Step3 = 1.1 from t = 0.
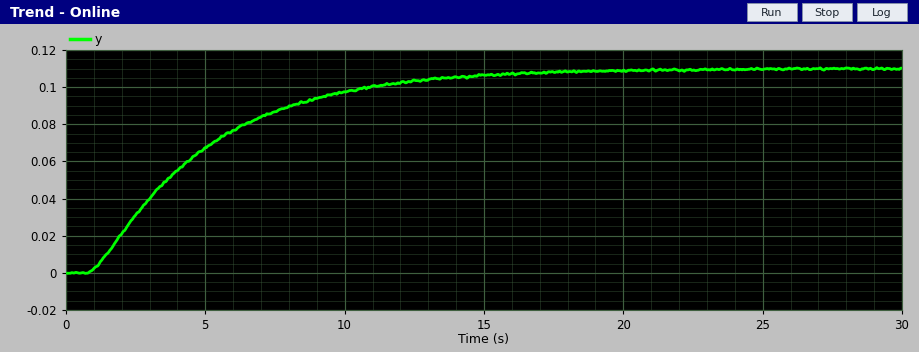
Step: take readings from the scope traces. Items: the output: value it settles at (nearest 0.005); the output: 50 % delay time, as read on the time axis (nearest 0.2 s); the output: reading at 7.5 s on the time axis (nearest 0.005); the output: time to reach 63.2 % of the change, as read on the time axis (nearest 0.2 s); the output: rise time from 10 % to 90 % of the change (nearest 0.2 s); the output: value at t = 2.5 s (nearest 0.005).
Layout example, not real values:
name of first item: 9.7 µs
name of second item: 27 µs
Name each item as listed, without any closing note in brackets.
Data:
the output: value it settles at: 0.110
the output: 50 % delay time, as read on the time axis: 4.0 s
the output: reading at 7.5 s on the time axis: 0.085
the output: time to reach 63.2 % of the change, as read on the time axis: 5.2 s
the output: rise time from 10 % to 90 % of the change: 9.0 s
the output: value at t = 2.5 s: 0.030
